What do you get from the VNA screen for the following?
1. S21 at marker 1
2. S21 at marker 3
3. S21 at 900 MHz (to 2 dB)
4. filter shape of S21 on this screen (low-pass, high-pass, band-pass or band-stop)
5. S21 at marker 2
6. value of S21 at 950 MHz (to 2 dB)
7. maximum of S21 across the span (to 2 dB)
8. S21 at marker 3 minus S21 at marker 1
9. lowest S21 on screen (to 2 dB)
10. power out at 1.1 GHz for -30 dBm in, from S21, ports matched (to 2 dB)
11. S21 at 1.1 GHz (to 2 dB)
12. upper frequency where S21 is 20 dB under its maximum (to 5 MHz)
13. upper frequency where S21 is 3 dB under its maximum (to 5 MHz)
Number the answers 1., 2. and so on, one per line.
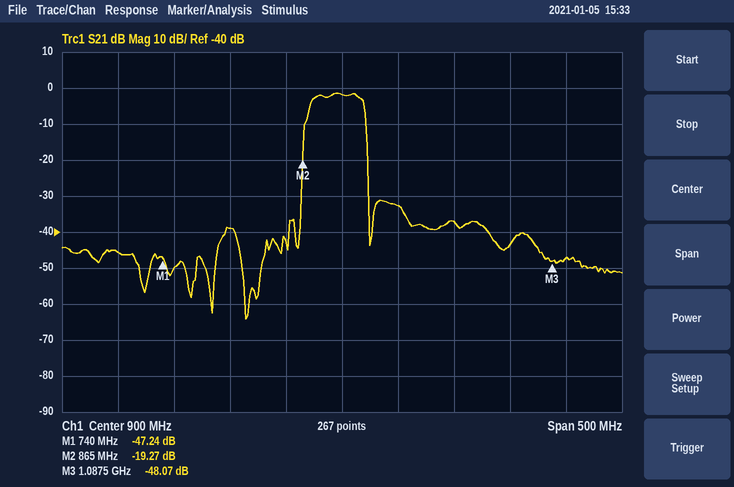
1. -47.24 dB
2. -48.07 dB
3. -2 dB
4. band-pass
5. -19.27 dB
6. -32 dB
7. -2 dB
8. -0.83 dB
9. -64 dB
10. -78 dBm
11. -48 dB
12. 925 MHz
13. 920 MHz
